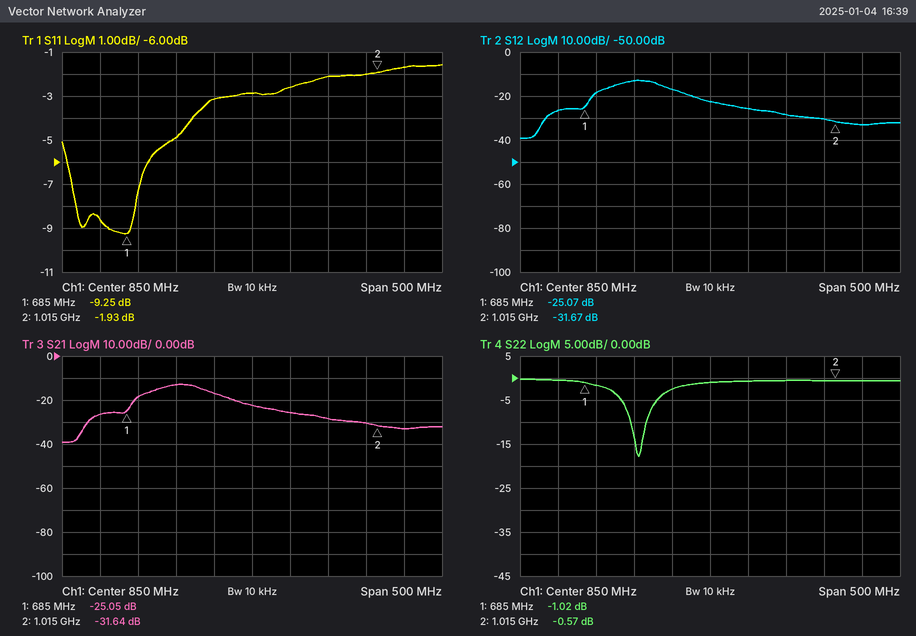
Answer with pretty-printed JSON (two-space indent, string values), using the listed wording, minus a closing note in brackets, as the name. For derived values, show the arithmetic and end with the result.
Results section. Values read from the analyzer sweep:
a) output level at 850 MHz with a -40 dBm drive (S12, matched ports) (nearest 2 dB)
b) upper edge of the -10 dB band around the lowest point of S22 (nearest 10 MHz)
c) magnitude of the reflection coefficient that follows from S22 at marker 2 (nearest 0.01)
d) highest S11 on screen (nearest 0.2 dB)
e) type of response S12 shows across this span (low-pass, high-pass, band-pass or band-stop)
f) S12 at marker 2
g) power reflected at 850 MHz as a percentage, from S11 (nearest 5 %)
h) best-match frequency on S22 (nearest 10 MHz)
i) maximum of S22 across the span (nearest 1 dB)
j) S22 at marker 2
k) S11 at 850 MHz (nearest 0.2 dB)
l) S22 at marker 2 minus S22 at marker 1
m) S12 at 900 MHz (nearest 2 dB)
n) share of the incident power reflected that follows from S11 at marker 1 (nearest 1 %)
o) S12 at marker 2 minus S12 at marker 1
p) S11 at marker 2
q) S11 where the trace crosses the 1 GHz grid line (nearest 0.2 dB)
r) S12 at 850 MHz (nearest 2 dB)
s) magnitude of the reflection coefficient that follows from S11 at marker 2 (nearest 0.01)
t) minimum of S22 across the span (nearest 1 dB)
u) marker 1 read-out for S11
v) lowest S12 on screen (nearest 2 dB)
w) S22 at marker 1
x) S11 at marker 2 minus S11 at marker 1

{
  "output level at 850 MHz with a -40 dBm drive (S12, matched ports)": "-40 dBm + (-22 dB) = -62 dBm",
  "upper edge of the -10 dB band around the lowest point of S22": "770 MHz",
  "magnitude of the reflection coefficient that follows from S22 at marker 2": "10^(-0.57/20) ≈ 0.94",
  "highest S11 on screen": "-1.6 dB",
  "type of response S12 shows across this span": "band-pass",
  "S12 at marker 2": "-31.67 dB",
  "power reflected at 850 MHz as a percentage, from S11": "10^(-2.8/10) ≈ 52.5 %, so 50 % to the nearest 5 %",
  "best-match frequency on S22": "760 MHz",
  "maximum of S22 across the span": "0 dB",
  "S22 at marker 2": "-0.57 dB",
  "S11 at 850 MHz": "-2.8 dB",
  "S22 at marker 2 minus S22 at marker 1": "-0.57 − (-1.02) = 0.45 dB",
  "S12 at 900 MHz": "-26 dB",
  "share of the incident power reflected that follows from S11 at marker 1": "10^(-9.25/10) ≈ 12 %",
  "S12 at marker 2 minus S12 at marker 1": "-31.67 − (-25.07) = -6.60 dB",
  "S11 at marker 2": "-1.93 dB",
  "S11 where the trace crosses the 1 GHz grid line": "-2.0 dB",
  "S12 at 850 MHz": "-22 dB",
  "magnitude of the reflection coefficient that follows from S11 at marker 2": "10^(-1.93/20) ≈ 0.80",
  "minimum of S22 across the span": "-18 dB",
  "marker 1 read-out for S11": "-9.25 dB",
  "lowest S12 on screen": "-40 dB",
  "S22 at marker 1": "-1.02 dB",
  "S11 at marker 2 minus S11 at marker 1": "-1.93 − (-9.25) = 7.32 dB"
}
